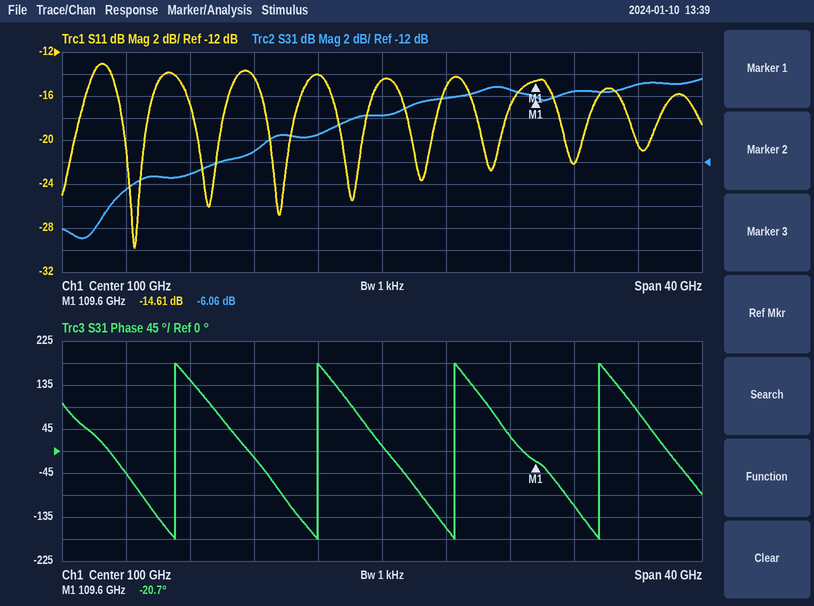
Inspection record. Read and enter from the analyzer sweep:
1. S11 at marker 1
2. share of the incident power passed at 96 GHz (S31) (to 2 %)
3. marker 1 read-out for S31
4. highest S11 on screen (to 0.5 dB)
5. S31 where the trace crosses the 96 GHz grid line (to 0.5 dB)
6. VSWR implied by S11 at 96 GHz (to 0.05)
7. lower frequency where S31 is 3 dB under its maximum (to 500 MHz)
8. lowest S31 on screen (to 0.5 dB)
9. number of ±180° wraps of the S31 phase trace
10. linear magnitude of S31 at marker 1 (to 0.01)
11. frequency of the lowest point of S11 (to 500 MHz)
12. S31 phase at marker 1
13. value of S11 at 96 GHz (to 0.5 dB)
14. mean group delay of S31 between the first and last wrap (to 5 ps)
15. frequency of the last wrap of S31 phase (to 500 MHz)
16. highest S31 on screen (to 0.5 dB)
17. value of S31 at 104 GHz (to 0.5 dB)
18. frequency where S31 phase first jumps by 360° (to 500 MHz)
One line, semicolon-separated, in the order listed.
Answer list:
-14.61 dB; 12 %; -6.06 dB; -13.0 dB; -9.5 dB; 1.50; 101.0 GHz; -19.0 dB; 4; 0.50; 84.5 GHz; -20.7°; -14.0 dB; 115 ps; 113.5 GHz; -4.5 dB; -6.0 dB; 87.0 GHz
